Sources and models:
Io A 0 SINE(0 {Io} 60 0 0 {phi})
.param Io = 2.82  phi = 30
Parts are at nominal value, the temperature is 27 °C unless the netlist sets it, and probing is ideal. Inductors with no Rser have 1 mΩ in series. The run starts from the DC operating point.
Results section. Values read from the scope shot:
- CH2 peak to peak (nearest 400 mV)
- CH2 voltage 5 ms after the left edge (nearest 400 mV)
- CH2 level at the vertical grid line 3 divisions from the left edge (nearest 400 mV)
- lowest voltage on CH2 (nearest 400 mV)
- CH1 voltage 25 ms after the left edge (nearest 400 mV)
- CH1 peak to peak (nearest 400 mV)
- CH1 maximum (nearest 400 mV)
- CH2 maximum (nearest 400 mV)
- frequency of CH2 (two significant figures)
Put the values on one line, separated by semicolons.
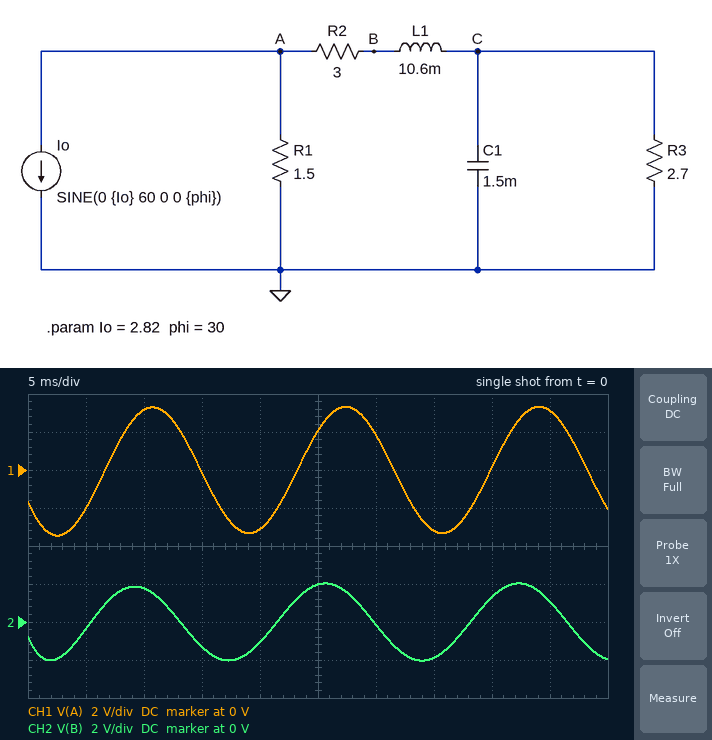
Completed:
4.0 V; -400 mV; -1.2 V; -2.0 V; 2.0 V; 6.8 V; 3.2 V; 2.0 V; 61 Hz
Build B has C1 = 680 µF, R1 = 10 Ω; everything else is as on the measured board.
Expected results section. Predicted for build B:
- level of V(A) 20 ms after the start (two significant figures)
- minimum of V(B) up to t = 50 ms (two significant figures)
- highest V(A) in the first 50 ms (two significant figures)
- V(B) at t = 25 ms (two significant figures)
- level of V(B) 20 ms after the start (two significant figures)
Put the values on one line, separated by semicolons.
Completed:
-8.9 V; -7.1 V; 10 V; 6.0 V; -3.3 V
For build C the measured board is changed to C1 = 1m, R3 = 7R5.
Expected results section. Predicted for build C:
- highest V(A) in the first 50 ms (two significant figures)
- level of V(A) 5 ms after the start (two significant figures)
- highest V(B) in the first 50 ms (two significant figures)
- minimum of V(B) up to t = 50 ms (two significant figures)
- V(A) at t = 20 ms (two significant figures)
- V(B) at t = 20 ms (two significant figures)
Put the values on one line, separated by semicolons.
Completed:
3.2 V; -2.2 V; 1.4 V; -2.6 V; -3.0 V; -730 mV
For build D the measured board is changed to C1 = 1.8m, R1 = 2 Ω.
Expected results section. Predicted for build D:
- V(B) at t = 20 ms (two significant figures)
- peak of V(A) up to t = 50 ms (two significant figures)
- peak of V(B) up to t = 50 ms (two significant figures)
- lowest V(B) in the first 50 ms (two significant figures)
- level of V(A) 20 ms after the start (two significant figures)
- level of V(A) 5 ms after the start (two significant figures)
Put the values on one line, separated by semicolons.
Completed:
-1.2 V; 4.1 V; 2.6 V; -2.6 V; -3.8 V; -2.4 V
